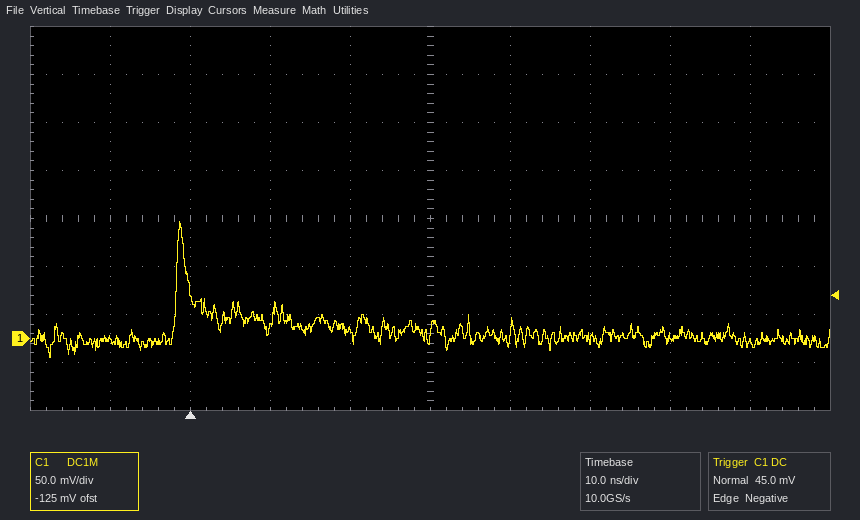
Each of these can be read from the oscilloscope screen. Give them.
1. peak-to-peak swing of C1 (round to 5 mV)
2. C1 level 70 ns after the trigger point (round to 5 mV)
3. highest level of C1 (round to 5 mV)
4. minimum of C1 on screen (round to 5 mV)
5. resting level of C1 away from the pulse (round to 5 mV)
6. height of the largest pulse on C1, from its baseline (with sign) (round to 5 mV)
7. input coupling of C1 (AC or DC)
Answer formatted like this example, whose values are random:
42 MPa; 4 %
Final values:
140 mV; -5 mV; 120 mV; -20 mV; 0 mV; +120 mV; DC
